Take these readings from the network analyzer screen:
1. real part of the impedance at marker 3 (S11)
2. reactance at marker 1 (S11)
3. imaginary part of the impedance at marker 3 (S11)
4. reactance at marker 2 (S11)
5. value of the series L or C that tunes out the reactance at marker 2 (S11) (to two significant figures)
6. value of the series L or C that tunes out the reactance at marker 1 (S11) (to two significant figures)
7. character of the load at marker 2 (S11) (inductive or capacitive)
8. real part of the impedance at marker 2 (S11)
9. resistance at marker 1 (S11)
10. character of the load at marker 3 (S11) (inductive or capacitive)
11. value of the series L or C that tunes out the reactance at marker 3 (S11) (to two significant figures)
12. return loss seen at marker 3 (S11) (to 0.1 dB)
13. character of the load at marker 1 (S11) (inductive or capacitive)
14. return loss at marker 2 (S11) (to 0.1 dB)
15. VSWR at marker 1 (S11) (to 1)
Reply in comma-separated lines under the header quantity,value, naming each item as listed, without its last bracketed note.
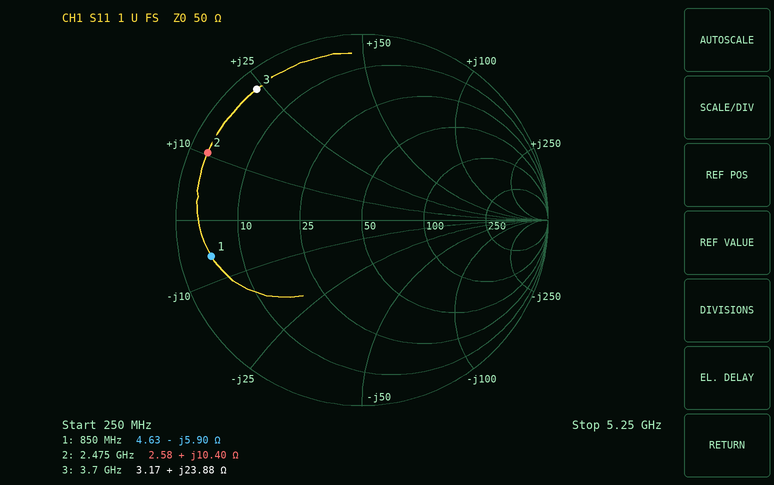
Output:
quantity,value
real part of the impedance at marker 3,3.17 Ω
reactance at marker 1,-5.90 Ω
imaginary part of the impedance at marker 3,+23.88 Ω
reactance at marker 2,+10.40 Ω
value of the series L or C that tunes out the reactance at marker 2 (S11),6.2 pF
value of the series L or C that tunes out the reactance at marker 1 (S11),1.1 nH
character of the load at marker 2 (S11),inductive
real part of the impedance at marker 2,2.58 Ω
resistance at marker 1,4.63 Ω
character of the load at marker 3 (S11),inductive
value of the series L or C that tunes out the reactance at marker 3 (S11),1.8 pF
return loss seen at marker 3 (S11),0.9 dB
character of the load at marker 1 (S11),capacitive
return loss at marker 2 (S11),0.9 dB
VSWR at marker 1 (S11),11
